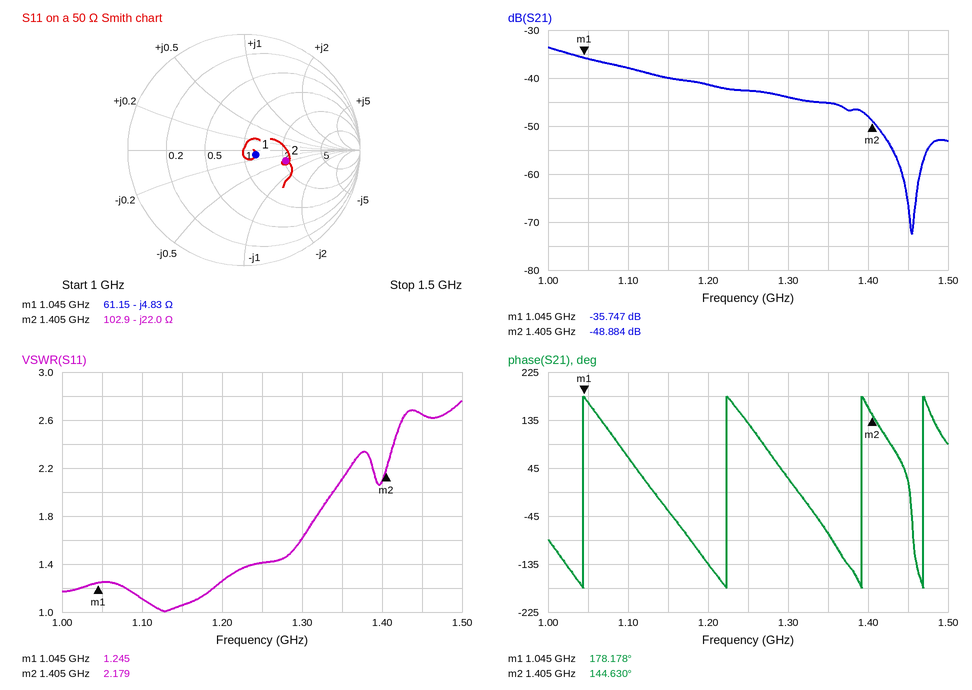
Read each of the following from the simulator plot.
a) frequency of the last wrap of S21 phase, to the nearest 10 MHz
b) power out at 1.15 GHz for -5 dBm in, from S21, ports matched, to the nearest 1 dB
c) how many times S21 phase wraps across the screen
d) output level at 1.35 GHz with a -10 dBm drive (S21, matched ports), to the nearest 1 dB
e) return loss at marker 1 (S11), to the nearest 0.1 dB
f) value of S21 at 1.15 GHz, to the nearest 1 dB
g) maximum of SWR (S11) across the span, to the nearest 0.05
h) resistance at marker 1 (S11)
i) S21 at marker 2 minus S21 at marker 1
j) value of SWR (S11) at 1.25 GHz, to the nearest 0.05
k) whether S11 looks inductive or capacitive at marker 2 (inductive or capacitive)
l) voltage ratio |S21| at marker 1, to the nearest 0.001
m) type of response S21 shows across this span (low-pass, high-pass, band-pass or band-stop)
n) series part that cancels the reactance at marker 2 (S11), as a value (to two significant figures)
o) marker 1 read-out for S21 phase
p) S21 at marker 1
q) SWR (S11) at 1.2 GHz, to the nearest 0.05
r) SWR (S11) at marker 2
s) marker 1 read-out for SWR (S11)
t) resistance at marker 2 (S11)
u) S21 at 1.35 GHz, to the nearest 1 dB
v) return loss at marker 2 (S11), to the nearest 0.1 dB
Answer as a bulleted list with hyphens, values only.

- 1.47 GHz
- -45 dBm
- 4
- -55 dBm
- 19.2 dB
- -40 dB
- 2.75
- 61.15 Ω
- -13.137 dB
- 1.40
- capacitive
- 0.016
- low-pass
- 2.5 nH
- 178.178°
- -35.747 dB
- 1.25
- 2.179
- 1.245
- 102.9 Ω
- -45 dB
- 8.6 dB
